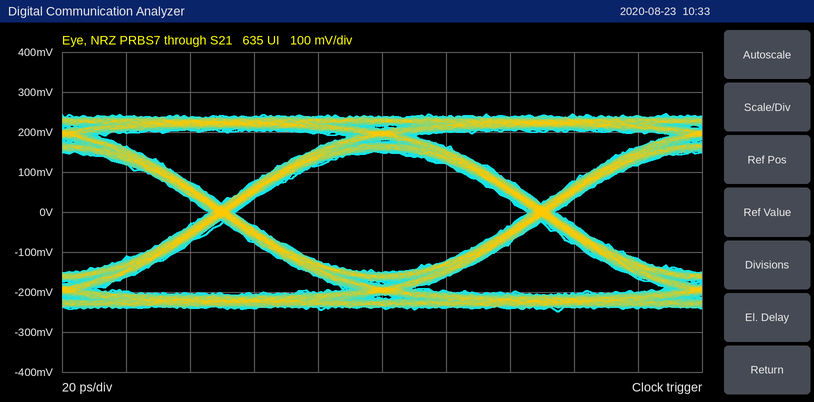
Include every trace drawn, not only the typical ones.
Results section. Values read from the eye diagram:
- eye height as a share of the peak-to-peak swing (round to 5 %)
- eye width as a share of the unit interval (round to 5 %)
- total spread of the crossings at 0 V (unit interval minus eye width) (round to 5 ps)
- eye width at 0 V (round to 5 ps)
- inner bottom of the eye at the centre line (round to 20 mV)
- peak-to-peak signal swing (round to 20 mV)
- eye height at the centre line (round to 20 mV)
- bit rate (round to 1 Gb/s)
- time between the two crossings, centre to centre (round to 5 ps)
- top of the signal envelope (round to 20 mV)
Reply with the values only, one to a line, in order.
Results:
60 %
90 %
10 ps
90 ps
-160 mV
500 mV
300 mV
10 Gb/s
100 ps
240 mV
